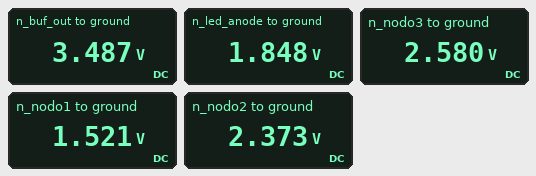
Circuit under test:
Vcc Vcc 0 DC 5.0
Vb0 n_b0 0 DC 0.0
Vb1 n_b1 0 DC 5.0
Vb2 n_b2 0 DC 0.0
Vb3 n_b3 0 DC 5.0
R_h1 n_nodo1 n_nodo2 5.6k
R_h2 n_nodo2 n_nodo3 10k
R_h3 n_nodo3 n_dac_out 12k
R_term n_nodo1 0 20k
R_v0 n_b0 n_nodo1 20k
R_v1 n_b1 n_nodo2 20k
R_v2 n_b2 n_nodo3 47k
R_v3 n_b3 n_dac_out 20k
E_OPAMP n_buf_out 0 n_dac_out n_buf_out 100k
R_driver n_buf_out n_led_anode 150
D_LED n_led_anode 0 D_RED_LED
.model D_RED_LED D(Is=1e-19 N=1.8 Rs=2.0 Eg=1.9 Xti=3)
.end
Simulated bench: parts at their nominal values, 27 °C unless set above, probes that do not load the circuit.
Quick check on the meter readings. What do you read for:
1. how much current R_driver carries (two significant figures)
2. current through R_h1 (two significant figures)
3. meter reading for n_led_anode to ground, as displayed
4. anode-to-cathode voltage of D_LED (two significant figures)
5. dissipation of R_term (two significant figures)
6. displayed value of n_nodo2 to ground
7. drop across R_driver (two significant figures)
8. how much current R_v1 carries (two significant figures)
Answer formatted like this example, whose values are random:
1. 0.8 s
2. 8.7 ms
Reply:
1. 11 mA
2. 150 µA
3. 1.848 V
4. 1.8 V
5. 120 µW
6. 2.373 V
7. 1.6 V
8. 130 µA
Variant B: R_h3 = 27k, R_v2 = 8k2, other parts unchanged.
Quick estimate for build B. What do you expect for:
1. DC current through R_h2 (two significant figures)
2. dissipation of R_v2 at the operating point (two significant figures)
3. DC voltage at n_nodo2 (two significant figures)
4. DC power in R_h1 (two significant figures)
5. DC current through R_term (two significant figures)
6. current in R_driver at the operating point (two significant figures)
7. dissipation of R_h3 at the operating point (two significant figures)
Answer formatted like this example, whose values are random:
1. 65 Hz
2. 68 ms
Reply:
1. 56 µA
2. 160 µW
3. 1.7 V
4. 66 µW
5. 54 µA
6. 10 mA
7. 180 µW
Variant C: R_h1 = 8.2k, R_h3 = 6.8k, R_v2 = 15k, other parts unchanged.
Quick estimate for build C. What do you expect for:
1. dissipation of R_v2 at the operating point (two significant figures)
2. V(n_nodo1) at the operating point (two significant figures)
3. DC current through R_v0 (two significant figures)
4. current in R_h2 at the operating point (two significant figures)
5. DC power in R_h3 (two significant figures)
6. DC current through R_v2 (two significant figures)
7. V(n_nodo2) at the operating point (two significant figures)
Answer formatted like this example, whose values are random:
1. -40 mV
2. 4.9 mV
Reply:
1. 260 µW
2. 1.2 V
3. 60 µA
4. 20 µA
5. 86 µW
6. 130 µA
7. 2.2 V
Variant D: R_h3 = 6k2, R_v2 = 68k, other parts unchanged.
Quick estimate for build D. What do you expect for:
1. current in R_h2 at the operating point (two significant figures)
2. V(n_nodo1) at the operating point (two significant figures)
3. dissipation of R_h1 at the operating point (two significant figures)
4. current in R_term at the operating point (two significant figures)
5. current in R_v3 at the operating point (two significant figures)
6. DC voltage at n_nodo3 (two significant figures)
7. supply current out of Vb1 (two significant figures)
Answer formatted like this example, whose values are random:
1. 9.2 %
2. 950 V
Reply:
1. 38 µA
2. 1.6 V
3. 150 µW
4. 81 µA
5. 80 µA
6. 2.9 V
7. 120 µA
